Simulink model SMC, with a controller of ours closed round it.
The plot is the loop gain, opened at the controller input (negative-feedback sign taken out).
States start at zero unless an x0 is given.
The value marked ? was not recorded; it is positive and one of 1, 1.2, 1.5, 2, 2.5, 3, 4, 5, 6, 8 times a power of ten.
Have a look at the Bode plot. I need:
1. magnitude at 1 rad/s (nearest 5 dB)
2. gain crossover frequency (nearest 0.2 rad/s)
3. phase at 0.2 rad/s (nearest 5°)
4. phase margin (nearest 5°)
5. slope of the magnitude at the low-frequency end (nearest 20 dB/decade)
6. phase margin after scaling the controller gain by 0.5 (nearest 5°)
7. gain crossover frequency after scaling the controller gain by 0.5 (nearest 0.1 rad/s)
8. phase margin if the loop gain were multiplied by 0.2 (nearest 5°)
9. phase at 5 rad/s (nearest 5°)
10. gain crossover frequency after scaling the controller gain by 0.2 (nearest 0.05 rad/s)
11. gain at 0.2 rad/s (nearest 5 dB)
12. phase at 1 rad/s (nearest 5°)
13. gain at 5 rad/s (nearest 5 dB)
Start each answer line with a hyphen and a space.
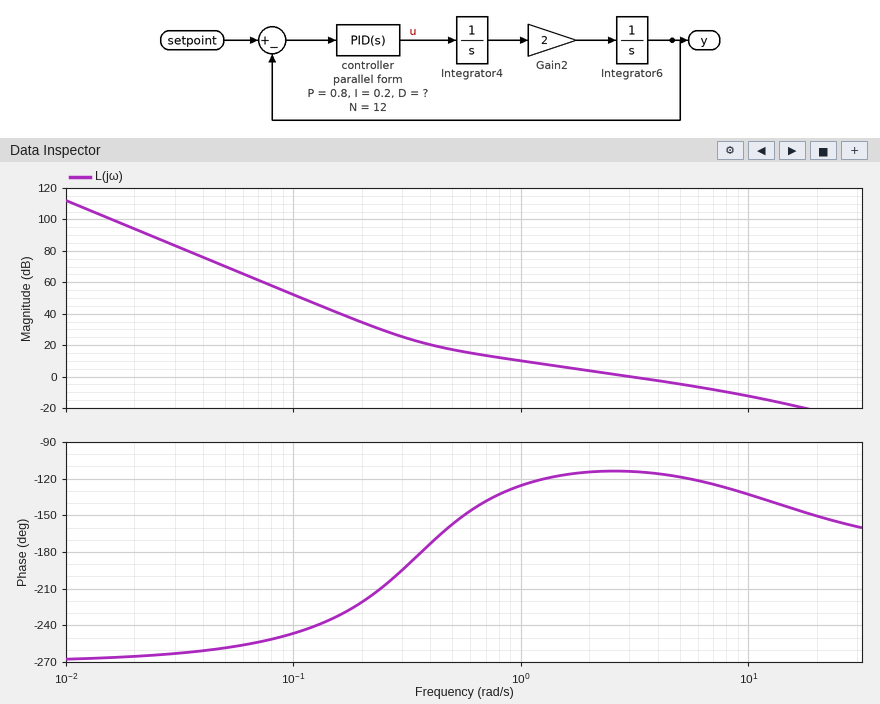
- 10 dB
- 3.0 rad/s
- -220°
- 65°
- -60 dB/decade
- 65°
- 1.6 rad/s
- 40°
- -120°
- 0.65 rad/s
- 35 dB
- -125°
- -5 dB
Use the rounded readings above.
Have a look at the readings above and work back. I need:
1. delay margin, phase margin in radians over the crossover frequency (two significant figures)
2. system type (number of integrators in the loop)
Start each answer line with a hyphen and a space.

- 0.38 s
- 3
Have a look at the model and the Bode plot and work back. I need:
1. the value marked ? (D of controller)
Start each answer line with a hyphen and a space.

- 1.5
